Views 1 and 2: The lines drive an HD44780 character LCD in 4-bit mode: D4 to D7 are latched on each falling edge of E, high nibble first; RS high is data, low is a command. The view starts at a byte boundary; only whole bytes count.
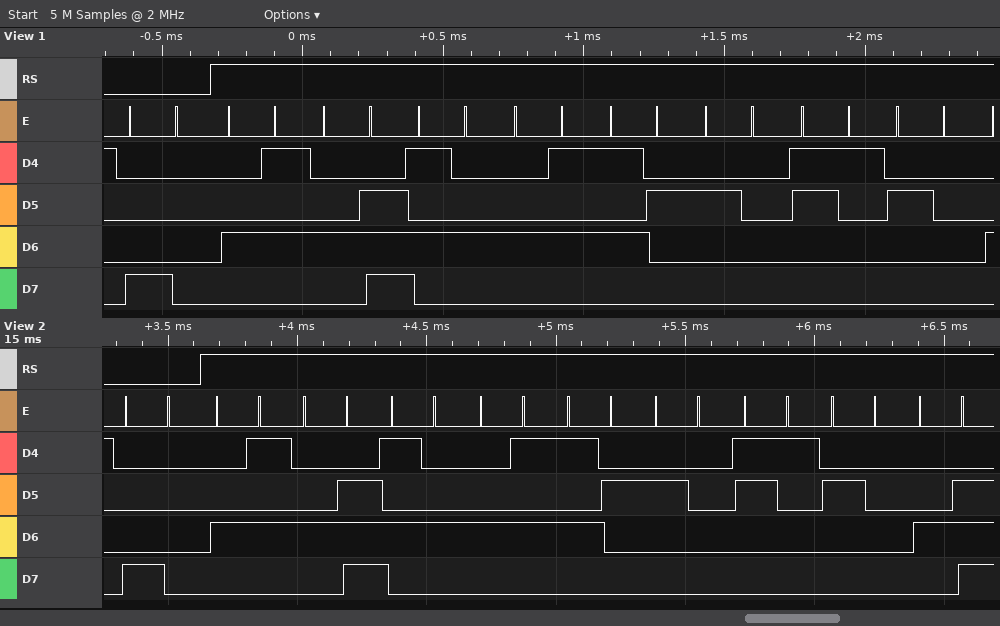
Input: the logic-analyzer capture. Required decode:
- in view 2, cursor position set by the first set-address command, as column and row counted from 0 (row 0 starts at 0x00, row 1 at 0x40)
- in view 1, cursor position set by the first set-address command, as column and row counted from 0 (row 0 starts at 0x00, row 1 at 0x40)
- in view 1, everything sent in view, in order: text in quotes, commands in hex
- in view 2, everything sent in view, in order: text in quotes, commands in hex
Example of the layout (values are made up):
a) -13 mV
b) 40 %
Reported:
a) column 0, row 0
b) column 0, row 0
c) 0x80 "ENTER 1 "
d) 0x80 "ENTER 1 N"
